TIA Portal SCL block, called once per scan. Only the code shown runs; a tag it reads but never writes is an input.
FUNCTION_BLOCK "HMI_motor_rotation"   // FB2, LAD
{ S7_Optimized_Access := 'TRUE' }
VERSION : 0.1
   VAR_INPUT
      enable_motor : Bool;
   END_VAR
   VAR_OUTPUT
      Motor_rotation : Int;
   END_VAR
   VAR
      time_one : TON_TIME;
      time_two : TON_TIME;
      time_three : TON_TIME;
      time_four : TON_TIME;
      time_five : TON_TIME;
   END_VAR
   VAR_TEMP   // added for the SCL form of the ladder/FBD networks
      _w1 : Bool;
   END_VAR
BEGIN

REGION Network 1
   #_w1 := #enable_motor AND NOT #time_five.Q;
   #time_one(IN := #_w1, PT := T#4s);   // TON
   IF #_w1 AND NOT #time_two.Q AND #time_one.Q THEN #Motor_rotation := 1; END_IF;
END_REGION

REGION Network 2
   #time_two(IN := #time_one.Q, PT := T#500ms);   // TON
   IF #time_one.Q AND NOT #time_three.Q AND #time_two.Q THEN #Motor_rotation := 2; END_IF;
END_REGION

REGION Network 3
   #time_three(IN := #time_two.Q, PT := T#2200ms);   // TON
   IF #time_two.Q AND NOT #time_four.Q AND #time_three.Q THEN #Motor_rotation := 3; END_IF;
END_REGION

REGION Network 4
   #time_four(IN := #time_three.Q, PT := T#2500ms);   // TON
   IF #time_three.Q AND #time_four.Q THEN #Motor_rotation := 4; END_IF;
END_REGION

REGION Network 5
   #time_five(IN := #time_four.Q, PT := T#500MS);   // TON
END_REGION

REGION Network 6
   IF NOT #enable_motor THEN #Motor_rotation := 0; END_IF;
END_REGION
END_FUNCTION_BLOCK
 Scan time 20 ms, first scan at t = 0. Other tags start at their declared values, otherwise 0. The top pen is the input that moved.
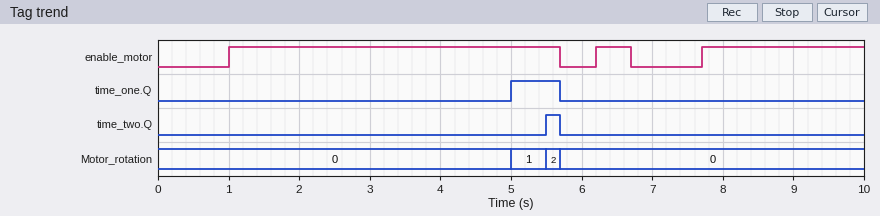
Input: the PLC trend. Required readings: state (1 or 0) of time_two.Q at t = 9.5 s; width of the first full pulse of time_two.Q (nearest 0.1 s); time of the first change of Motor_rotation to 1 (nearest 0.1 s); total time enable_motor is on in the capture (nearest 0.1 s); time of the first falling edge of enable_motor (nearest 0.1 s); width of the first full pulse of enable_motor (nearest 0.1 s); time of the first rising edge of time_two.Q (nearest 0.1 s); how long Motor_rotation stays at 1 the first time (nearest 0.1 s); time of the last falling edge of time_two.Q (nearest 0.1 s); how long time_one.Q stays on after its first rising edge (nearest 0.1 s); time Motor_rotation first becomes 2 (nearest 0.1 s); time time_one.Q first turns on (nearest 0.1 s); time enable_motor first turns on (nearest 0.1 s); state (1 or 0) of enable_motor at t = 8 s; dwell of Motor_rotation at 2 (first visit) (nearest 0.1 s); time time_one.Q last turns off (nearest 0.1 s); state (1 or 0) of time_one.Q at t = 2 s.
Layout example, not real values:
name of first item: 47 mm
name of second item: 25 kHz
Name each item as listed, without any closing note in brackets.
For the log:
state (1 or 0) of time_two.Q at t = 9.5 s: 0
width of the first full pulse of time_two.Q: 0.2 s
time of the first change of Motor_rotation to 1: 5.0 s
total time enable_motor is on in the capture: 7.5 s
time of the first falling edge of enable_motor: 5.7 s
width of the first full pulse of enable_motor: 4.7 s
time of the first rising edge of time_two.Q: 5.5 s
how long Motor_rotation stays at 1 the first time: 0.5 s
time of the last falling edge of time_two.Q: 5.7 s
how long time_one.Q stays on after its first rising edge: 0.7 s
time Motor_rotation first becomes 2: 5.5 s
time time_one.Q first turns on: 5.0 s
time enable_motor first turns on: 1.0 s
state (1 or 0) of enable_motor at t = 8 s: 1
dwell of Motor_rotation at 2 (first visit): 0.2 s
time time_one.Q last turns off: 5.7 s
state (1 or 0) of time_one.Q at t = 2 s: 0
